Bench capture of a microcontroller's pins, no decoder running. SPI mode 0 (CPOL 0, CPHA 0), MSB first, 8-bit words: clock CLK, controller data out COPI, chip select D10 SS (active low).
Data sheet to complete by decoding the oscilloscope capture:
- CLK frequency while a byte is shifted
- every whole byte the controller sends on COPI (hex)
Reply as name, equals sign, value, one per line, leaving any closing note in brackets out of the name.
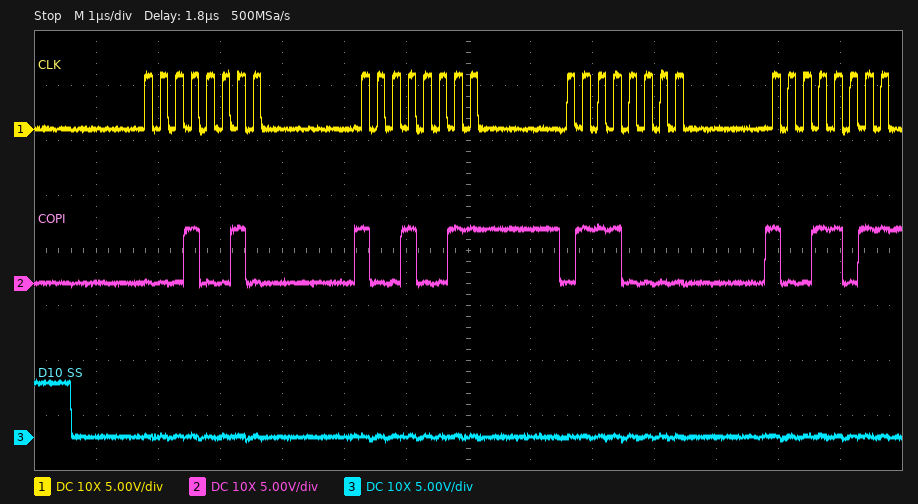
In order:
CLK frequency while a byte is shifted = 4 MHz
every whole byte the controller sends on COPI = 12 93 70 9B
